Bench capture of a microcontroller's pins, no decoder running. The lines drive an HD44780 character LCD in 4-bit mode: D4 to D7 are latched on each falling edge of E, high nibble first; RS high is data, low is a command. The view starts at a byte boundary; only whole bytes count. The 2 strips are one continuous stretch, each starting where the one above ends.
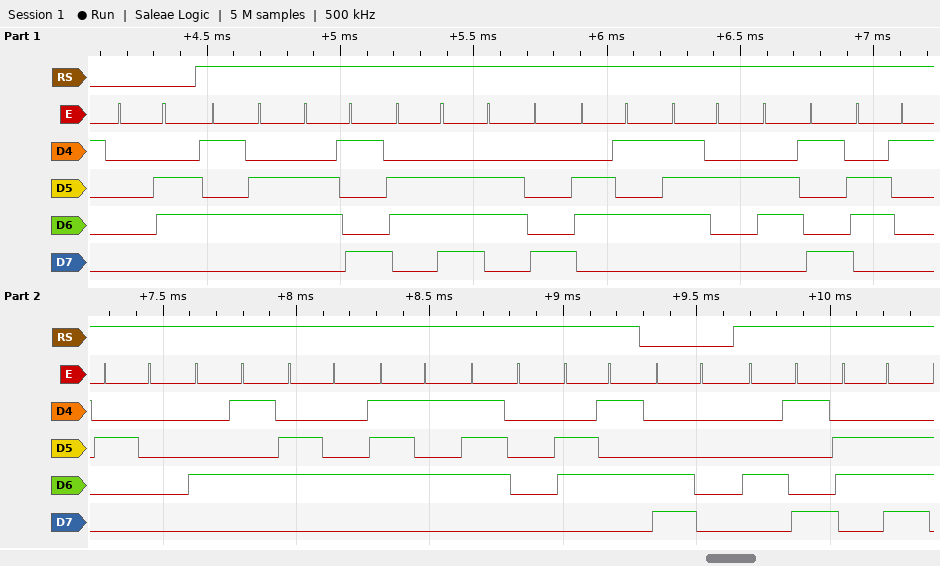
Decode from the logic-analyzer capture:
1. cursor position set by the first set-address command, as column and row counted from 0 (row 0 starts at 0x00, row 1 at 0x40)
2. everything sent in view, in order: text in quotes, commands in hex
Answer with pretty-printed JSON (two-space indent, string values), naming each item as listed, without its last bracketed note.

{
  "cursor position set by the first set-address command, as column and row counted from 0": "column 0, row 1",
  "everything sent in view, in order: text in quotes, commands in hex": "0x06 \"Vinheria Edupe\" 0xC0 \"In\""
}
